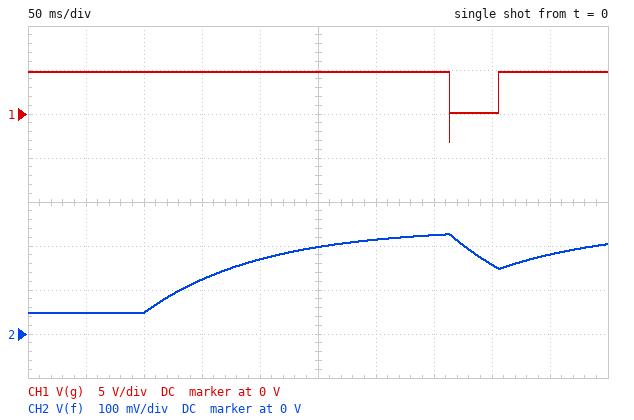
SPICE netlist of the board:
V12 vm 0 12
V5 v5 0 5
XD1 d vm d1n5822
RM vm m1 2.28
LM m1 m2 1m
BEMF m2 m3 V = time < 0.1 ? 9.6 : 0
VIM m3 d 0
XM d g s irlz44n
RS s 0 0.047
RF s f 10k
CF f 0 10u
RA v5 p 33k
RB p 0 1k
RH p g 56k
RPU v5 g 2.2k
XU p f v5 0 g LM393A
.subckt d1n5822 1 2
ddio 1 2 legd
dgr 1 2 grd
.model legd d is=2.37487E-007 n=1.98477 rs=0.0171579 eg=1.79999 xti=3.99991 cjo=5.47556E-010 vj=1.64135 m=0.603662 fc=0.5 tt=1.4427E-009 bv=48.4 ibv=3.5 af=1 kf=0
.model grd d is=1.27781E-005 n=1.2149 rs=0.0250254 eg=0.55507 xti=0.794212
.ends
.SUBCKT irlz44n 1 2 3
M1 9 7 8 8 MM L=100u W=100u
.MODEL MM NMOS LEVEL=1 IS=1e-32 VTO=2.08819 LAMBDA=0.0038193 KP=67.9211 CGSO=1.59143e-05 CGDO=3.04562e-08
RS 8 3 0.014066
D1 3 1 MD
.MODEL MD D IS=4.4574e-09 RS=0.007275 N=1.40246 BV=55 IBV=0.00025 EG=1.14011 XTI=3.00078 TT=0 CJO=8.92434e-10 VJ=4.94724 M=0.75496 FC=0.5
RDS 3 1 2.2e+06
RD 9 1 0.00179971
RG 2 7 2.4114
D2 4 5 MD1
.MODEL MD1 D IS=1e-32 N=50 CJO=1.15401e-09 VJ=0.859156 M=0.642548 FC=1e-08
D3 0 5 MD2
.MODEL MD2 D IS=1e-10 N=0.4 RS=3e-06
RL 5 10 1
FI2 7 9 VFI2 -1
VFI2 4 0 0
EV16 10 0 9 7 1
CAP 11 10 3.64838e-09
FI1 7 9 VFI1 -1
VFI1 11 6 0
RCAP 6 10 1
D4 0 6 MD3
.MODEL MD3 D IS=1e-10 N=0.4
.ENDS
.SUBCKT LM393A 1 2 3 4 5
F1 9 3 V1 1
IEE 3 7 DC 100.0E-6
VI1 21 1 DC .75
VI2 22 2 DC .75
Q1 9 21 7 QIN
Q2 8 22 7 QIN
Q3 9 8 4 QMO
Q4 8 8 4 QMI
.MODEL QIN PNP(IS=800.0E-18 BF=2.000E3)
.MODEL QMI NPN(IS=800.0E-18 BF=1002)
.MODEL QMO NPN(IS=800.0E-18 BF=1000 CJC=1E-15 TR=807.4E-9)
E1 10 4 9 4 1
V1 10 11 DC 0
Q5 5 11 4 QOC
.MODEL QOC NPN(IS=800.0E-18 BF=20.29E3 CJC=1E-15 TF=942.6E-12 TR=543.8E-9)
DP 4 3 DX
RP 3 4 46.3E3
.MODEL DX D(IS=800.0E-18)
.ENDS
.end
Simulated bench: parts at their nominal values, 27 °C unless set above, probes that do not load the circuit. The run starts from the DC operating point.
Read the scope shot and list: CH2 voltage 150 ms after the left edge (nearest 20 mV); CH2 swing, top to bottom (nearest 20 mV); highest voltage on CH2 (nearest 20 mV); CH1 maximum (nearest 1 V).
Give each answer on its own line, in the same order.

120 mV
180 mV
220 mV
5 V
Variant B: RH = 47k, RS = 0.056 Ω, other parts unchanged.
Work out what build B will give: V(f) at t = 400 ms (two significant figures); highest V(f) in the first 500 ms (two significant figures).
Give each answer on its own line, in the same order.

230 mV
240 mV
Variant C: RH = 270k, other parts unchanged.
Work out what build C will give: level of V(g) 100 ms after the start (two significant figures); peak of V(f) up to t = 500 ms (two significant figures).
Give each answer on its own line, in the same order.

5.0 V
160 mV
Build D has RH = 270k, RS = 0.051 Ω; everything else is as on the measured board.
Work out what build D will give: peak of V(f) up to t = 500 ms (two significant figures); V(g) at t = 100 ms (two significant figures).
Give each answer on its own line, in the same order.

160 mV
5.0 V
